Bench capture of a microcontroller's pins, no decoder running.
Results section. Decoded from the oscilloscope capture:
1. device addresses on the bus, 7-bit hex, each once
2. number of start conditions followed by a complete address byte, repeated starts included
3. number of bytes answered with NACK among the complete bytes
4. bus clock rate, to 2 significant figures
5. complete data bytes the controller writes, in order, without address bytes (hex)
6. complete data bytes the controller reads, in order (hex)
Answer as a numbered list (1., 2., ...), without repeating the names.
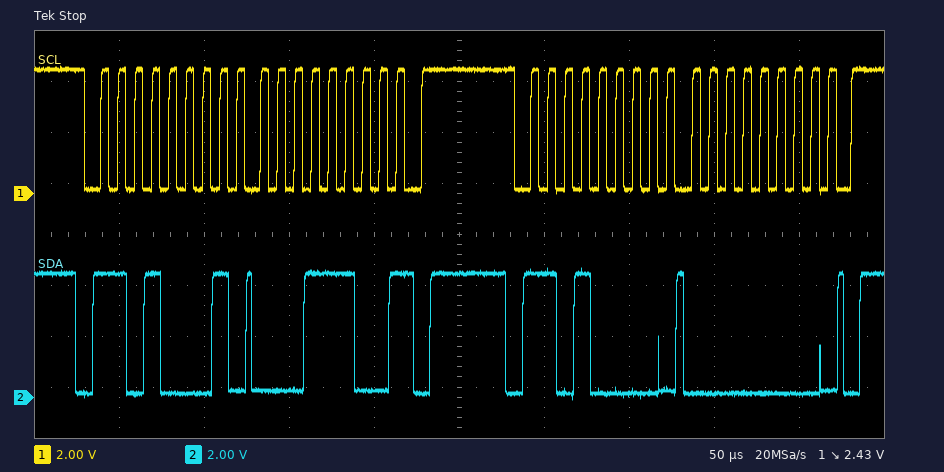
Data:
1. 0x68
2. 2
3. 1
4. 100 kHz
5. 00
6. 1C
